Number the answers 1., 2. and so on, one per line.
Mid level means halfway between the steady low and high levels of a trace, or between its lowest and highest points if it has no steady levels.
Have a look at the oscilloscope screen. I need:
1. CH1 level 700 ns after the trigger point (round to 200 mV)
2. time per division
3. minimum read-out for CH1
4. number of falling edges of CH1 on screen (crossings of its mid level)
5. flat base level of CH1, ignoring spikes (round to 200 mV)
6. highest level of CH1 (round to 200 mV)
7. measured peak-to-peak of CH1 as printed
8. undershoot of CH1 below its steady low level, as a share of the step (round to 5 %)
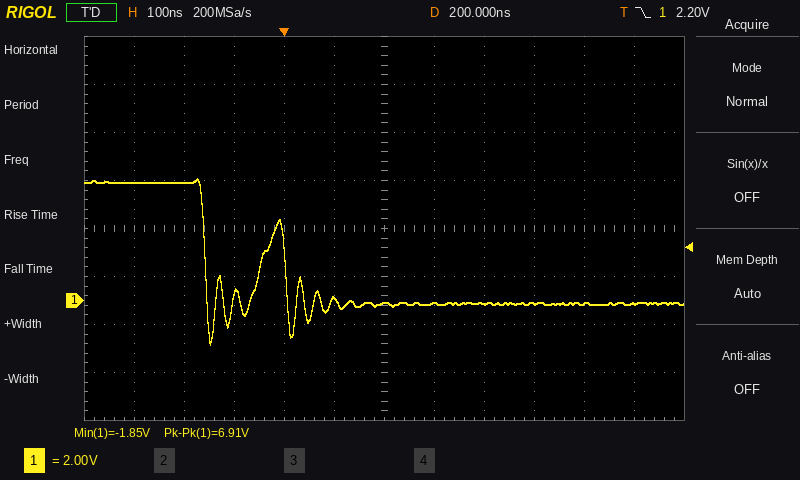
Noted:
1. -200 mV
2. 100 ns
3. -1.85 V
4. 2
5. -200 mV
6. 5.0 V
7. 6.91 V
8. 35 %
